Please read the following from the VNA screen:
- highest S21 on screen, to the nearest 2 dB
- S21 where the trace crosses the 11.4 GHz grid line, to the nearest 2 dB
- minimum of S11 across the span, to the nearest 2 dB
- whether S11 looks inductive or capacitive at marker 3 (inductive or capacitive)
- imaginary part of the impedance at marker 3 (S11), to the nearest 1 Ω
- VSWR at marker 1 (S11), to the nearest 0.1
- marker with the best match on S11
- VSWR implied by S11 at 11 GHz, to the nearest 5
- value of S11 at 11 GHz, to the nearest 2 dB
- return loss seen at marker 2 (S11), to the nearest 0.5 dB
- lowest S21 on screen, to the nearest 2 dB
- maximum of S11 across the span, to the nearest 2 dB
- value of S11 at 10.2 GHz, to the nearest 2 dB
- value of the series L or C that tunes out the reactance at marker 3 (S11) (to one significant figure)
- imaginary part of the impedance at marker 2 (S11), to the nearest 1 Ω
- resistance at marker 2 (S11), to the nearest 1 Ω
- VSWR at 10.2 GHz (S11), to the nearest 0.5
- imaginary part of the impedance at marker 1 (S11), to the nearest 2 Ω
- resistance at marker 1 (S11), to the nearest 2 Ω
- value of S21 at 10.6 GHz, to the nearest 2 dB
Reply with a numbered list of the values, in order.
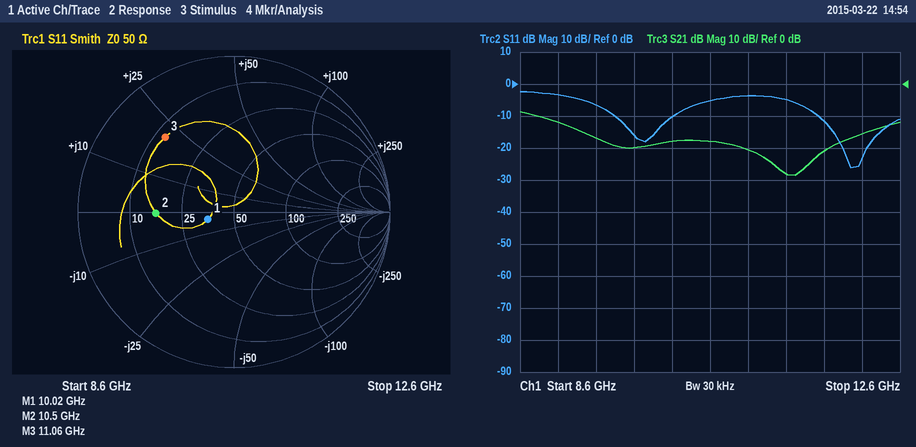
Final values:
1. -8 dB
2. -28 dB
3. -26 dB
4. inductive
5. +21 Ω
6. 1.4
7. marker 1
8. 5
9. -4 dB
10. 6.0 dB
11. -28 dB
12. -2 dB
13. -10 dB
14. 700 fF
15. 0 Ω
16. 17 Ω
17. 2.0
18. -4 Ω
19. 36 Ω
20. -18 dB
